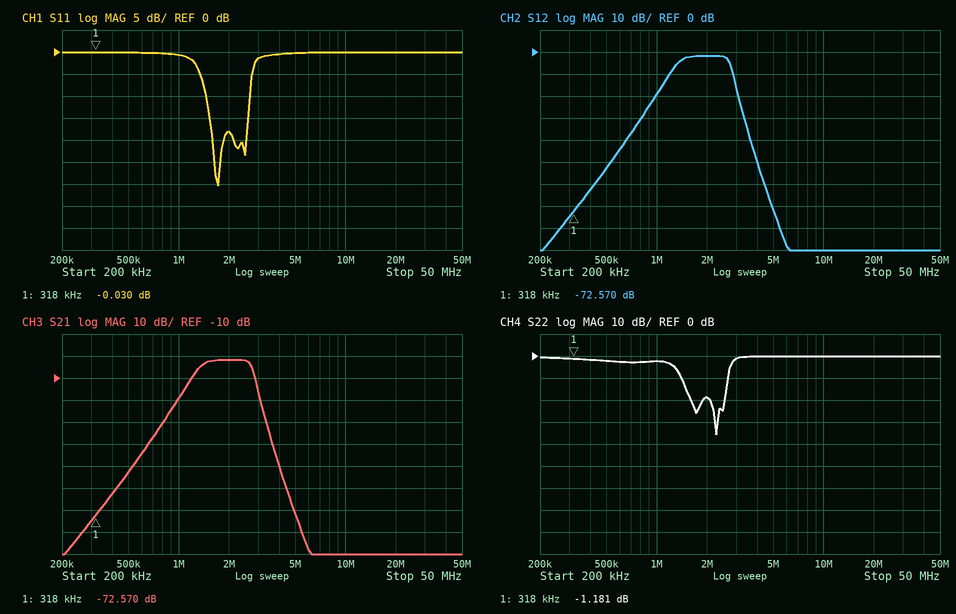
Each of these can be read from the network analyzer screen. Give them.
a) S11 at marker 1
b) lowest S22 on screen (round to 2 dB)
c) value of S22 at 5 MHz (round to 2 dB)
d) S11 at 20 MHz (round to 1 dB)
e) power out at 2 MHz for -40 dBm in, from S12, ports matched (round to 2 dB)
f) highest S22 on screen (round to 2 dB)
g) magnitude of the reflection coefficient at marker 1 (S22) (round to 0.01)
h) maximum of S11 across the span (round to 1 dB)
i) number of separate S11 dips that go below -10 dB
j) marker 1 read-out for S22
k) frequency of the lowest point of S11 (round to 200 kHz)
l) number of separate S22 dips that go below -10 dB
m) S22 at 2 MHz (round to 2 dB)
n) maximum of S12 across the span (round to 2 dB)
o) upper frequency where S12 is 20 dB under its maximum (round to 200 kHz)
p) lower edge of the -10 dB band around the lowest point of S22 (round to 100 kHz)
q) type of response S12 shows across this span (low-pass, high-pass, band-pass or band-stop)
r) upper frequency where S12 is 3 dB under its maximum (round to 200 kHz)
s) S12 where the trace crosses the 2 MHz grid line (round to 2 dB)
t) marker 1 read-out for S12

-0.030 dB
-36 dB
0 dB
0 dB
-42 dBm
0 dB
0.87
0 dB
2
-1.181 dB
1.8 MHz
2
-18 dB
-2 dB
3.2 MHz
1.4 MHz
band-pass
2.8 MHz
-2 dB
-72.570 dB
